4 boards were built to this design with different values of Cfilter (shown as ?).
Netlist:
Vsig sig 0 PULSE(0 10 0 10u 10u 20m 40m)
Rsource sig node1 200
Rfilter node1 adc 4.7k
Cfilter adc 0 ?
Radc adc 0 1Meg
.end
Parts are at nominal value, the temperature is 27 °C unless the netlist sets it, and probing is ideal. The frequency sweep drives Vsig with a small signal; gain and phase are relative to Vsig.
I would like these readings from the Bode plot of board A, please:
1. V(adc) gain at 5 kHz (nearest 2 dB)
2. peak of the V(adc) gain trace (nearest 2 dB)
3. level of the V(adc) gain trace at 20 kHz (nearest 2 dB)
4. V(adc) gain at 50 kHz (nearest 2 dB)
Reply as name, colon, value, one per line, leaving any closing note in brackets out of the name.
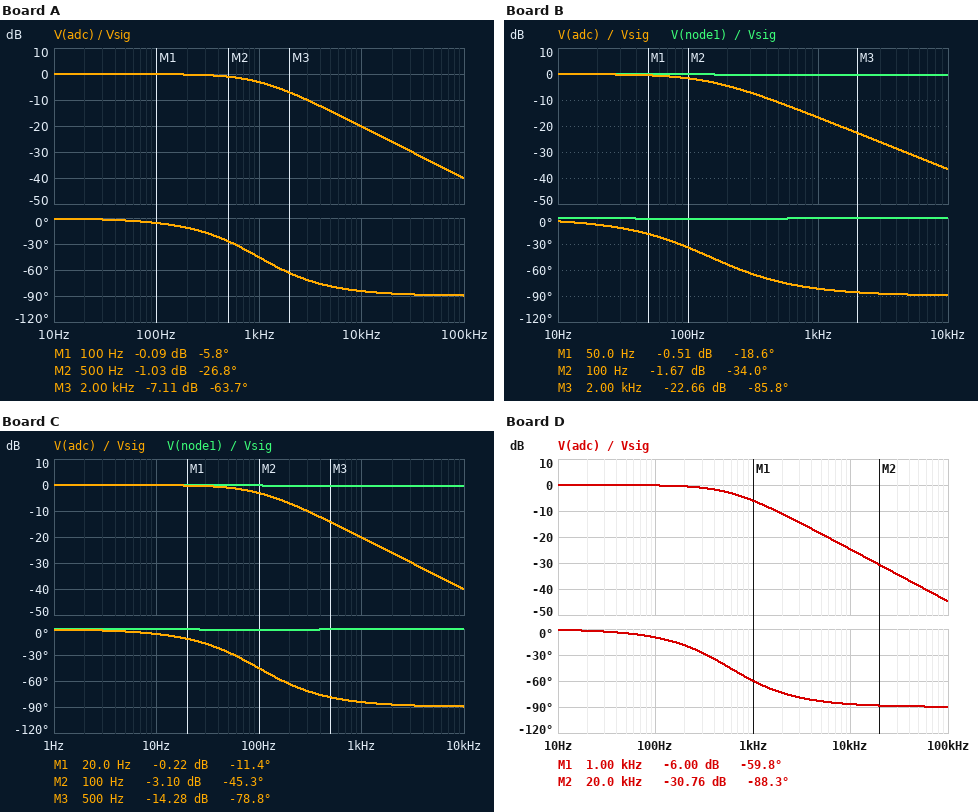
V(adc) gain at 5 kHz: -14 dB
peak of the V(adc) gain trace: 0 dB
level of the V(adc) gain trace at 20 kHz: -26 dB
V(adc) gain at 50 kHz: -34 dB
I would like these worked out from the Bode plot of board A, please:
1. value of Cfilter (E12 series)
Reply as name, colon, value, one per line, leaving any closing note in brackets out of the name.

value of Cfilter: 33 nF
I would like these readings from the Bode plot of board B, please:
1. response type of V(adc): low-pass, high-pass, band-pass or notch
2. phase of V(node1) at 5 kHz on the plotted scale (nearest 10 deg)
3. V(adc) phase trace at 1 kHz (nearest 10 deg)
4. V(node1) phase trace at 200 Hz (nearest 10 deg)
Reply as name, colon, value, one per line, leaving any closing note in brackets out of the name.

response type of V(adc): low-pass, high-pass, band-pass or notch: low-pass
phase of V(node1) at 5 kHz on the plotted scale: 0 deg
V(adc) phase trace at 1 kHz: -80 deg
V(node1) phase trace at 200 Hz: 0 deg
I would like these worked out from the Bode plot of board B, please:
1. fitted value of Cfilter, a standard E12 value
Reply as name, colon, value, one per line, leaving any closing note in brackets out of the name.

fitted value of Cfilter, a standard E12 value: 220 nF
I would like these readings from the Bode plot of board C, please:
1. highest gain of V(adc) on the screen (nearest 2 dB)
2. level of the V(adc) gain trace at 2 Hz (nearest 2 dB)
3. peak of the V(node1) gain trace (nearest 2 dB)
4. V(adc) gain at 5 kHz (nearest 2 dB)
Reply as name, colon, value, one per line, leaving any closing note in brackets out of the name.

highest gain of V(adc) on the screen: 0 dB
level of the V(adc) gain trace at 2 Hz: 0 dB
peak of the V(node1) gain trace: 0 dB
V(adc) gain at 5 kHz: -34 dB
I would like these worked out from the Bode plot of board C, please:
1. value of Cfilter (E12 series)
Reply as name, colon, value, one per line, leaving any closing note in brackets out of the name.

value of Cfilter: 330 nF
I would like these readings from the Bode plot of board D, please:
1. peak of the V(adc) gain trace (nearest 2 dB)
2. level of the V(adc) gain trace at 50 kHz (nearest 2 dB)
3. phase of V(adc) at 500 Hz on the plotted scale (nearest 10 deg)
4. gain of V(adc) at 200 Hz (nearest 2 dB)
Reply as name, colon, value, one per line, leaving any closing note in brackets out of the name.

peak of the V(adc) gain trace: 0 dB
level of the V(adc) gain trace at 50 kHz: -38 dB
phase of V(adc) at 500 Hz on the plotted scale: -40 deg
gain of V(adc) at 200 Hz: 0 dB
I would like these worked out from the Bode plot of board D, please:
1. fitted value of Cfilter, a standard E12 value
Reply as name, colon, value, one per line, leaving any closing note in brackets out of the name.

fitted value of Cfilter, a standard E12 value: 56 nF
